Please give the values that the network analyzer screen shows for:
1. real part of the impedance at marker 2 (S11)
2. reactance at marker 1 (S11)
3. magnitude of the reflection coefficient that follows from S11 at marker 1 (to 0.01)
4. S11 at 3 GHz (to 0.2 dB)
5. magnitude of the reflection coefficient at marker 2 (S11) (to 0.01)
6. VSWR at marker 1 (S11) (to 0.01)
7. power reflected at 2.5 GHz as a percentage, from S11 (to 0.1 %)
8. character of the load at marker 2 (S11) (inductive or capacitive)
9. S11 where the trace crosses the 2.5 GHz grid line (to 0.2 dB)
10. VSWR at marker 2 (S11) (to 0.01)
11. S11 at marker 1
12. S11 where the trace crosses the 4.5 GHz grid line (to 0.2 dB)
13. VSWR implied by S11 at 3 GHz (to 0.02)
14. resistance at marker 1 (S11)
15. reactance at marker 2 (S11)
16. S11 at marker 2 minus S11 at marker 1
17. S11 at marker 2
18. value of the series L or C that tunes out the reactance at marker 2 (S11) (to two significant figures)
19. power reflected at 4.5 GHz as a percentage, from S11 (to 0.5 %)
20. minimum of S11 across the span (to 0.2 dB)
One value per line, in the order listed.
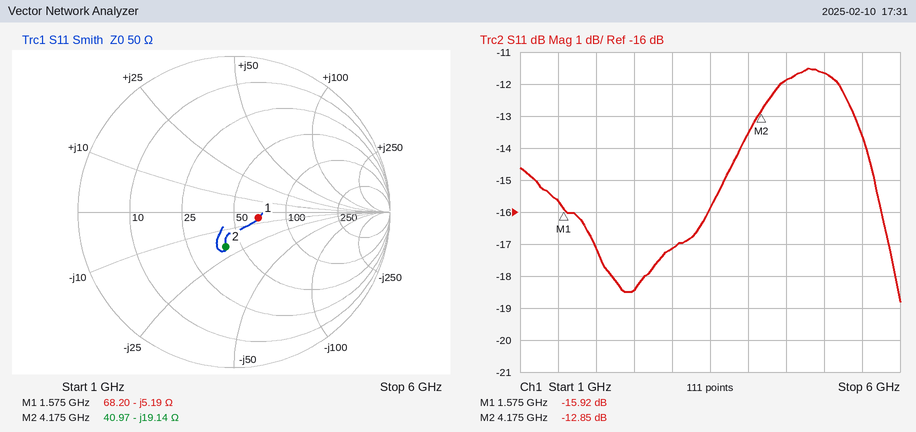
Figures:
40.97 Ω
-5.19 Ω
0.16
-17.2 dB
0.23
1.38
1.4 %
capacitive
-18.4 dB
1.59
-15.92 dB
-11.8 dB
1.32
68.20 Ω
-19.14 Ω
3.07 dB
-12.85 dB
730 pH
6.5 %
-18.8 dB
